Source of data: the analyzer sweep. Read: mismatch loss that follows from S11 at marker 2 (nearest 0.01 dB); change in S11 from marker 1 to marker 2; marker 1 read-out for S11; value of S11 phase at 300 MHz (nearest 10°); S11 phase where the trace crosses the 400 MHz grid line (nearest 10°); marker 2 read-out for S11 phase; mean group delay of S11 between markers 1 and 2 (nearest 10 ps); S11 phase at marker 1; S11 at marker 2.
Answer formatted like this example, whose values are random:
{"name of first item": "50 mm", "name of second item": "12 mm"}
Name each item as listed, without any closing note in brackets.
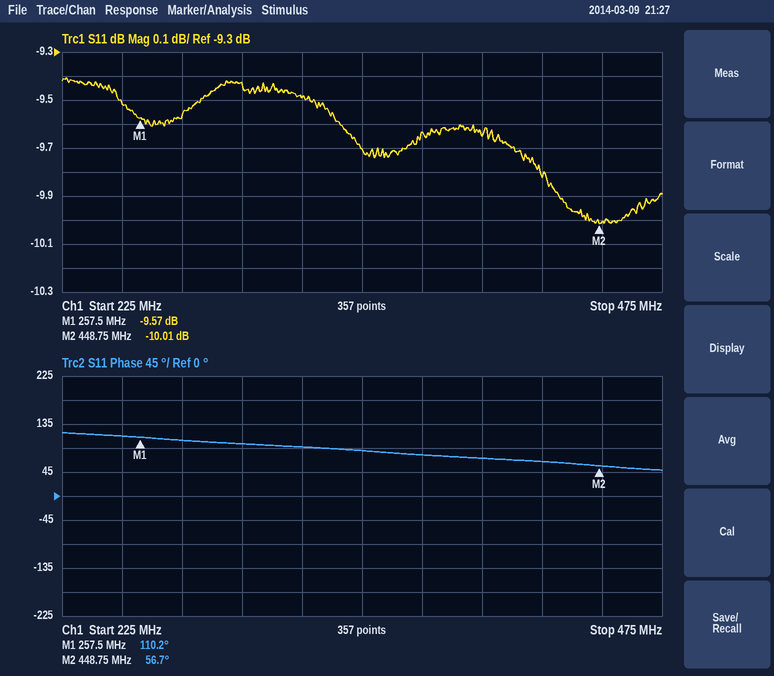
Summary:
{"mismatch loss that follows from S11 at marker 2": "0.46 dB", "change in S11 from marker 1 to marker 2": "-0.44 dB", "marker 1 read-out for S11": "-9.57 dB", "value of S11 phase at 300 MHz": "100°", "S11 phase where the trace crosses the 400 MHz grid line": "70°", "marker 2 read-out for S11 phase": "56.7°", "mean group delay of S11 between markers 1 and 2": "780 ps", "S11 phase at marker 1": "110.2°", "S11 at marker 2": "-10.01 dB"}
